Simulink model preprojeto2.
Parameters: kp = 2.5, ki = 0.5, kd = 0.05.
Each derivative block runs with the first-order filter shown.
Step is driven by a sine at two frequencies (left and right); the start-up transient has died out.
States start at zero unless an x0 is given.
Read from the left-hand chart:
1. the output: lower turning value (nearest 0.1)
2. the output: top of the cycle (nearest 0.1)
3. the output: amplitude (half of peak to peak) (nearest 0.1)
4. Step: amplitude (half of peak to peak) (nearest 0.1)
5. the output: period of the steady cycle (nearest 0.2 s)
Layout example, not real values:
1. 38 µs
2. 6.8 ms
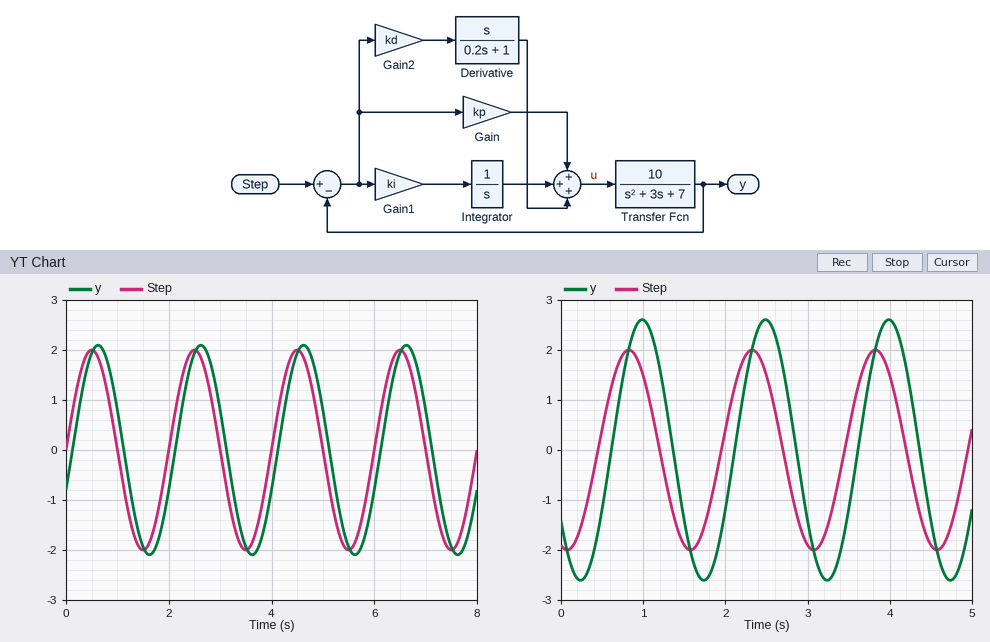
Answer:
1. -2.1
2. 2.1
3. 2.1
4. 2.0
5. 2.0 s
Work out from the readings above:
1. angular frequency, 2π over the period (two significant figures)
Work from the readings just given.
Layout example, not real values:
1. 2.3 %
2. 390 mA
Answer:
1. 3.1 rad/s
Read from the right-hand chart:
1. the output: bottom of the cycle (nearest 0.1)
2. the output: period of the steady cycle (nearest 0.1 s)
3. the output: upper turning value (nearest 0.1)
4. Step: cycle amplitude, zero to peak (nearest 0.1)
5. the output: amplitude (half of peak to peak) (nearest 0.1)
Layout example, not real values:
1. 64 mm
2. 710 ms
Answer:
1. -2.6
2. 1.5 s
3. 2.6
4. 2.0
5. 2.6
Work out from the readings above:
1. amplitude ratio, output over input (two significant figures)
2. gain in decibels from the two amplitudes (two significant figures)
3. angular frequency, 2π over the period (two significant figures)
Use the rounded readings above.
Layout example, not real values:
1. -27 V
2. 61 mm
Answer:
1. 1.3
2. 2.3 dB
3. 4.2 rad/s
